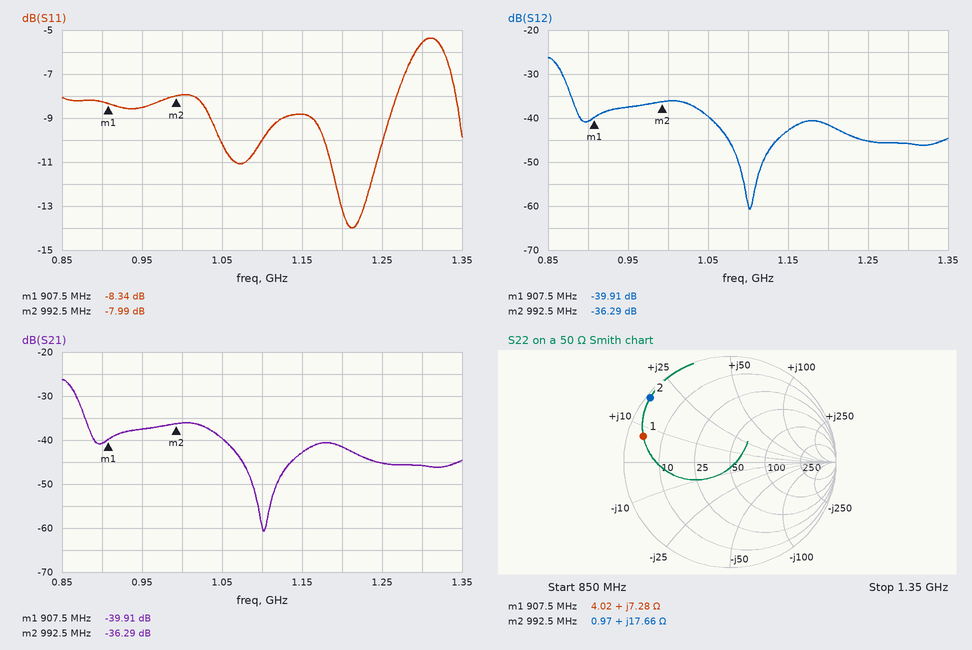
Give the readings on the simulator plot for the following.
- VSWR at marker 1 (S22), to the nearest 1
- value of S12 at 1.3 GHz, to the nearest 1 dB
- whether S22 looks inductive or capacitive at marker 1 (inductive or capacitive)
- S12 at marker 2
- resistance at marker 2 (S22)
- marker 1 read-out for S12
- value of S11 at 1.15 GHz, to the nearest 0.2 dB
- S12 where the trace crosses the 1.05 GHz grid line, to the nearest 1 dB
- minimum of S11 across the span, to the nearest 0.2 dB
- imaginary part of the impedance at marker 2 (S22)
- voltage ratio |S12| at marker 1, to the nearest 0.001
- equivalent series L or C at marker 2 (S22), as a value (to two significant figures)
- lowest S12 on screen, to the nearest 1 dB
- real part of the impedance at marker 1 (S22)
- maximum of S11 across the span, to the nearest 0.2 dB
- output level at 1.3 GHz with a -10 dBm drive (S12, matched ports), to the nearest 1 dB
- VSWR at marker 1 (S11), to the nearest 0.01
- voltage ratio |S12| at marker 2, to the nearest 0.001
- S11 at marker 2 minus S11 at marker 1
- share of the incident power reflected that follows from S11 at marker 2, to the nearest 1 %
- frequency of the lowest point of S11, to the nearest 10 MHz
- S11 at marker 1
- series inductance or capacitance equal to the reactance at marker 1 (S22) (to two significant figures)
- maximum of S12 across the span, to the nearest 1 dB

13
-46 dB
inductive
-36.29 dB
0.97 Ω
-39.91 dB
-8.8 dB
-40 dB
-14.0 dB
+17.66 Ω
0.010
2.8 nH
-61 dB
4.02 Ω
-5.4 dB
-56 dBm
2.24
0.015
0.35 dB
16 %
1.21 GHz
-8.34 dB
1.3 nH
-26 dB
